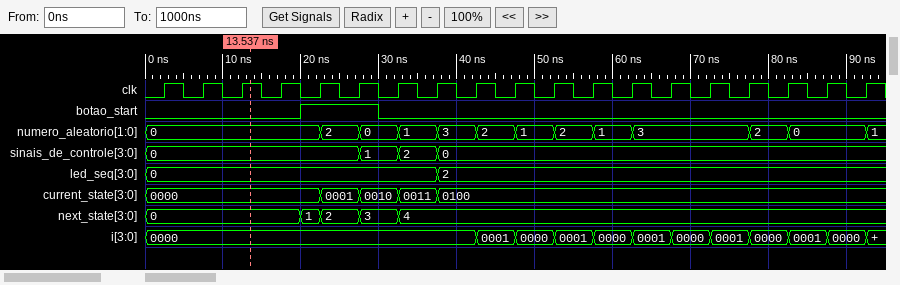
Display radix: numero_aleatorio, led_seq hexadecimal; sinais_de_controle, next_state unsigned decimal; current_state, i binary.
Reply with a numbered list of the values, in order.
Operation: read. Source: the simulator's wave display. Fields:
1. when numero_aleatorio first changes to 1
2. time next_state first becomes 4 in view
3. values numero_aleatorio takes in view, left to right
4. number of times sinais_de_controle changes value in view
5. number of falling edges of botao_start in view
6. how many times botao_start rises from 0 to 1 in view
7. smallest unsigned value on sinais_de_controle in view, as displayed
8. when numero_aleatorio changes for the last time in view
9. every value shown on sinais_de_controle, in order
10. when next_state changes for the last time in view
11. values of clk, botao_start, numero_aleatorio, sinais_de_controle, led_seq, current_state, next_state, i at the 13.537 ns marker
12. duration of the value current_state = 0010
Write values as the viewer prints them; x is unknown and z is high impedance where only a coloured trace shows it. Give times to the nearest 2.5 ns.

1. 32.5 ns
2. 32.5 ns
3. 0, 2, 0, 1, 3, 2, 1, 2, 1, 3, 2, 0, 1
4. 3
5. 1
6. 1
7. 0
8. 92.5 ns
9. 0, 1, 2, 0
10. 32.5 ns
11. clk=1, botao_start=0, numero_aleatorio=0, sinais_de_controle=0, led_seq=0, current_state=0000, next_state=0, i=0000
12. 5 ns
